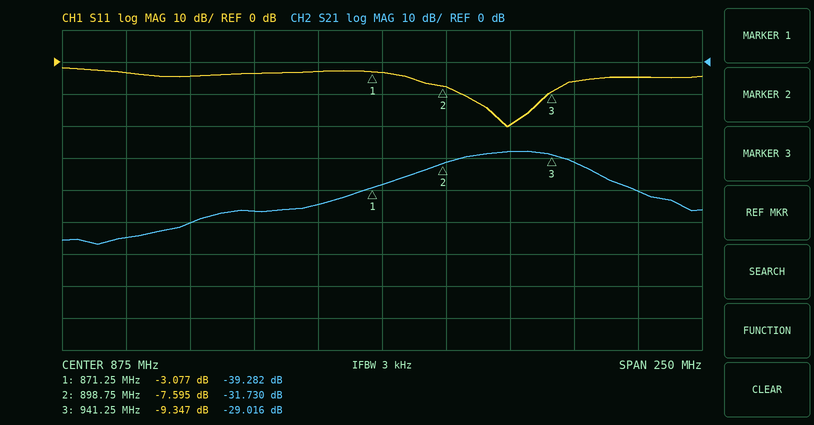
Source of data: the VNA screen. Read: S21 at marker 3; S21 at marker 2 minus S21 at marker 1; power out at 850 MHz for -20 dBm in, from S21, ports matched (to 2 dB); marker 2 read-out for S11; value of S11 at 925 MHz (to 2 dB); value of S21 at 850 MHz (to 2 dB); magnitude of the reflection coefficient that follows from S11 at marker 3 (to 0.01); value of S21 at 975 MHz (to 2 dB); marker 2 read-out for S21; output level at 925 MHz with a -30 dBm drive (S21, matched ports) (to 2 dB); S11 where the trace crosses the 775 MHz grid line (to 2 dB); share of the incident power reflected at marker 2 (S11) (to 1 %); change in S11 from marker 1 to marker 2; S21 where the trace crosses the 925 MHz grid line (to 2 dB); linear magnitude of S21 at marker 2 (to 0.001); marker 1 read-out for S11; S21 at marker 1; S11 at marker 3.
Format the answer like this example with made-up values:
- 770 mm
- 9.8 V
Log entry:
- -29.016 dB
- 7.552 dB
- -64 dBm
- -7.595 dB
- -20 dB
- -44 dB
- 0.34
- -40 dB
- -31.730 dB
- -58 dBm
- -4 dB
- 17 %
- -4.518 dB
- -28 dB
- 0.026
- -3.077 dB
- -39.282 dB
- -9.347 dB
